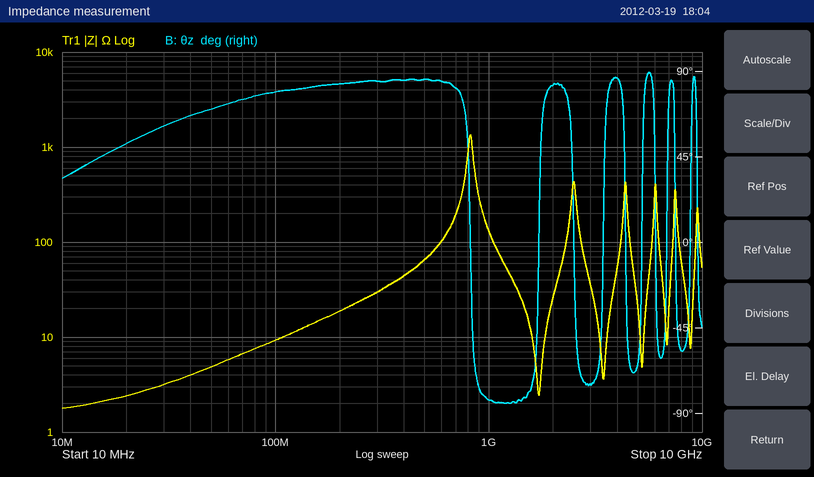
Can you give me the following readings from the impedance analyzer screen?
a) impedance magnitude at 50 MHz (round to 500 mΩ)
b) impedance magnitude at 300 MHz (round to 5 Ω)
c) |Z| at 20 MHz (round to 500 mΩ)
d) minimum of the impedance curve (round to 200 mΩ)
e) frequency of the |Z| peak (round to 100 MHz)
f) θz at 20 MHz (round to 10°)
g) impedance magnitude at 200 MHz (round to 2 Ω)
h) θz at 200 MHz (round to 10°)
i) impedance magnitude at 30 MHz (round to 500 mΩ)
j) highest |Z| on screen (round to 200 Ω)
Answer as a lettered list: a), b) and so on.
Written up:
a) 5.0 Ω
b) 30 Ω
c) 2.5 Ω
d) 1.8 Ω
e) 800 MHz
f) 50°
g) 18 Ω
h) 80°
i) 3.0 Ω
j) 1.4 kΩ
